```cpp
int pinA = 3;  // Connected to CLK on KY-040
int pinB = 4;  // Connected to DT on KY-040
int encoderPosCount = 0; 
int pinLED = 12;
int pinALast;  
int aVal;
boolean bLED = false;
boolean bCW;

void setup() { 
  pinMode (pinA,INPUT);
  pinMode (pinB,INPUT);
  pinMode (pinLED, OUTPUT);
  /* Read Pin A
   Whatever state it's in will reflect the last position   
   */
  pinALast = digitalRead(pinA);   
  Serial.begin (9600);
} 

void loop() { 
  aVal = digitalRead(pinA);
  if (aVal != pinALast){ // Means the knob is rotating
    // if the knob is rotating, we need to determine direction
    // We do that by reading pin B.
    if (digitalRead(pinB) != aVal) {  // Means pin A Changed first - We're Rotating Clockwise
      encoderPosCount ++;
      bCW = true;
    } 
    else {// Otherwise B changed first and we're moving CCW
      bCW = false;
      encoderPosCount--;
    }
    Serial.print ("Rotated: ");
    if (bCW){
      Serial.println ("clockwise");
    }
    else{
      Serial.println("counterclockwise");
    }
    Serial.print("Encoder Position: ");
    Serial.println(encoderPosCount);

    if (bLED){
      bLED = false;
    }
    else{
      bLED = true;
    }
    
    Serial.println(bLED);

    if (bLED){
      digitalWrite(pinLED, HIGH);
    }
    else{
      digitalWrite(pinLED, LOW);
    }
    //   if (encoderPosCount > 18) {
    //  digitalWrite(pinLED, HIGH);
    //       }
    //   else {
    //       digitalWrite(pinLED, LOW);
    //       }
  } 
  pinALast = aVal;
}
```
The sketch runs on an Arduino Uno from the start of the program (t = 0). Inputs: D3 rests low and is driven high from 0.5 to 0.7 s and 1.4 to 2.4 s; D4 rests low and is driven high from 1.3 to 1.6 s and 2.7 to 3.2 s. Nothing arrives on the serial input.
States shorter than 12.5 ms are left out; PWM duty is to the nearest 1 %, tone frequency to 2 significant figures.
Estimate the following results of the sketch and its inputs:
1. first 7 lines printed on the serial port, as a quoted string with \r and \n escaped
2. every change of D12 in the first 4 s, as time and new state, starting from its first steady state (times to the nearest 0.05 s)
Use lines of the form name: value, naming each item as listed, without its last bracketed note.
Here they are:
first 7 lines printed on the serial port, as a quoted string with \r and \n escaped: "Rotated: clockwise\r\nEncoder Position: 1\r\n1\r\nRotated: counterclockwise\r\nEncoder Position: 0\r\n0\r\nRotated: counterclockwise\r\n"
every change of D12 in the first 4 s, as time and new state, starting from its first steady state: 0 s low; 0.5 s high; 0.7 s low; 1.4 s high; 2.4 s low
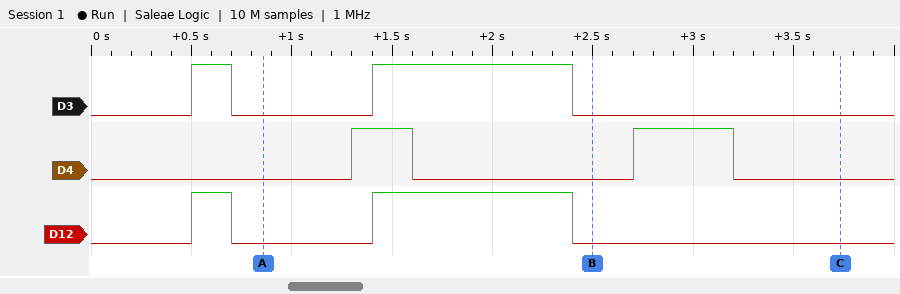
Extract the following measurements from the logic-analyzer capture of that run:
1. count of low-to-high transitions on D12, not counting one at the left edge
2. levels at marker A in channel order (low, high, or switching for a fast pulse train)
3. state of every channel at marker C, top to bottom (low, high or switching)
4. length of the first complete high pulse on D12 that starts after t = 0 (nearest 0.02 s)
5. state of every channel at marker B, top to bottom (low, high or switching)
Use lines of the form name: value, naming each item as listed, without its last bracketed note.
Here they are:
count of low-to-high transitions on D12, not counting one at the left edge: 2
levels at marker A in channel order: D3 low, D4 low, D12 low
state of every channel at marker C, top to bottom: D3 low, D4 low, D12 low
length of the first complete high pulse on D12 that starts after t = 0: 0.20 s
state of every channel at marker B, top to bottom: D3 low, D4 low, D12 low
